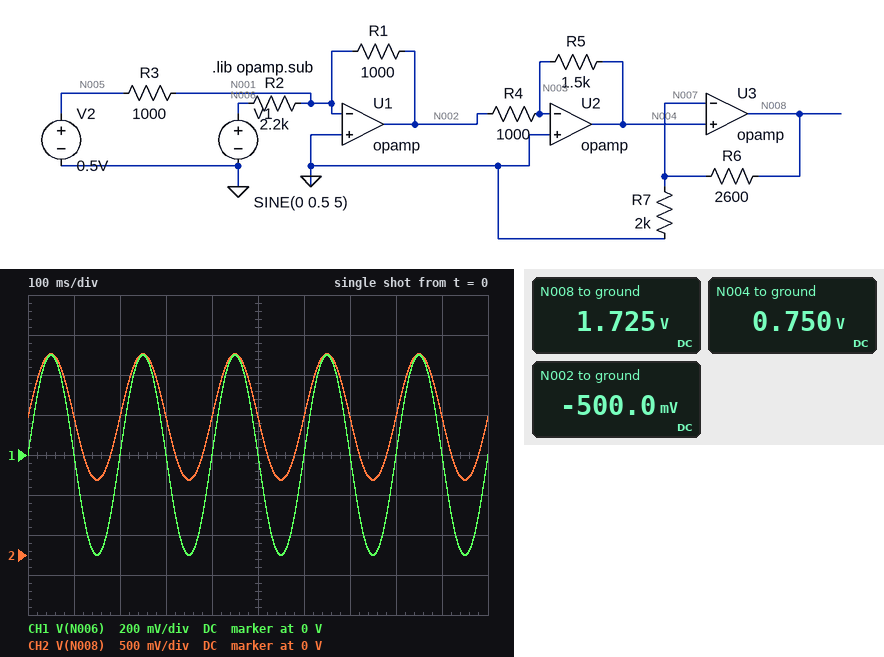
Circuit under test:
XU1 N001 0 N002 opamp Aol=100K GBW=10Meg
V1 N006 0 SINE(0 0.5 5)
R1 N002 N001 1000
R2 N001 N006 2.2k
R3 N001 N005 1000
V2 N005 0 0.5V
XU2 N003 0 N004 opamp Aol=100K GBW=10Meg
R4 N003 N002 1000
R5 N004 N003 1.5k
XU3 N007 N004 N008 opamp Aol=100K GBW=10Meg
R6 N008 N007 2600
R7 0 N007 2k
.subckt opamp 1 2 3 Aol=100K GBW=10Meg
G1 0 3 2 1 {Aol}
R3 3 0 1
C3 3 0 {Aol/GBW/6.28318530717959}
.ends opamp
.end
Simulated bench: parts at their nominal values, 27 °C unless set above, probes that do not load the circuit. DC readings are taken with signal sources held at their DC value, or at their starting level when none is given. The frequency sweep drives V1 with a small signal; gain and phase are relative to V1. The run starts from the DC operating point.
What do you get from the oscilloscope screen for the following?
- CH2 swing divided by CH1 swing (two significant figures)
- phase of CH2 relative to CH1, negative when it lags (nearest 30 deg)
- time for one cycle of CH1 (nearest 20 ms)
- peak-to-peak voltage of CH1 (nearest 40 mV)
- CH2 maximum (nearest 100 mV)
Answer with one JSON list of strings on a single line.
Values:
["1.6", "0 deg", "200 ms", "1.00 V", "2.5 V"]
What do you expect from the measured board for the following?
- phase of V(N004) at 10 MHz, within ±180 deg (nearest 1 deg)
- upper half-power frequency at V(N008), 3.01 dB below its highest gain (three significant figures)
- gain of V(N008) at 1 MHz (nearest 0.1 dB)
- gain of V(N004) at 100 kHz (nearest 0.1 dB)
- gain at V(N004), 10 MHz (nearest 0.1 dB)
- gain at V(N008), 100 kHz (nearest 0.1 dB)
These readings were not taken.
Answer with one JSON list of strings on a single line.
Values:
["-136 deg", "2.11 MHz", "3.2 dB", "-3.3 dB", "-20.4 dB", "3.9 dB"]
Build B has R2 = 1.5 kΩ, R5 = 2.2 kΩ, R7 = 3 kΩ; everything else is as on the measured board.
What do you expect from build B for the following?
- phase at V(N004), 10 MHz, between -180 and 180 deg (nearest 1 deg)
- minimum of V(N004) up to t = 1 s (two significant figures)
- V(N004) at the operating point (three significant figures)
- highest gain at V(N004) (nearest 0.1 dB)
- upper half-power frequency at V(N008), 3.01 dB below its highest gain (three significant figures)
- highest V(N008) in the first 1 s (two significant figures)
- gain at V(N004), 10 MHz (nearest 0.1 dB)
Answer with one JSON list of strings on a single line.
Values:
["-142 deg", "370 mV", "1.10 V", "3.3 dB", "1.95 MHz", "3.4 V", "-16.3 dB"]
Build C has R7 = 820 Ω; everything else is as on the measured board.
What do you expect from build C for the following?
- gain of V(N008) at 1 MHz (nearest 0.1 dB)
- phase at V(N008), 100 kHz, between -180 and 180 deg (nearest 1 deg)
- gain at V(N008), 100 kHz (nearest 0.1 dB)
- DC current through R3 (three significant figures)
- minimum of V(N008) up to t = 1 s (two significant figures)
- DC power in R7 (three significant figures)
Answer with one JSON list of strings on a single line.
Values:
["7.9 dB", "-5 deg", "9.1 dB", "500 µA", "1.7 V", "686 µW"]
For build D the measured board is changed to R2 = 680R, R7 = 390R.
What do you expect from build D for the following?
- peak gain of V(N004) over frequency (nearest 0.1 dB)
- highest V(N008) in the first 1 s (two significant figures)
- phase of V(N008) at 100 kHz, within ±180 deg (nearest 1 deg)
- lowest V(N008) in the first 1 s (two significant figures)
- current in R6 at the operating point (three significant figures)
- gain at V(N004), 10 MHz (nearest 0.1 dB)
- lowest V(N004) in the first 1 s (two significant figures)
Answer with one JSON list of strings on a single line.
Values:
["6.9 dB", "14 V", "-8 deg", "-2.7 V", "1.92 mA", "-12.9 dB", "-350 mV"]
